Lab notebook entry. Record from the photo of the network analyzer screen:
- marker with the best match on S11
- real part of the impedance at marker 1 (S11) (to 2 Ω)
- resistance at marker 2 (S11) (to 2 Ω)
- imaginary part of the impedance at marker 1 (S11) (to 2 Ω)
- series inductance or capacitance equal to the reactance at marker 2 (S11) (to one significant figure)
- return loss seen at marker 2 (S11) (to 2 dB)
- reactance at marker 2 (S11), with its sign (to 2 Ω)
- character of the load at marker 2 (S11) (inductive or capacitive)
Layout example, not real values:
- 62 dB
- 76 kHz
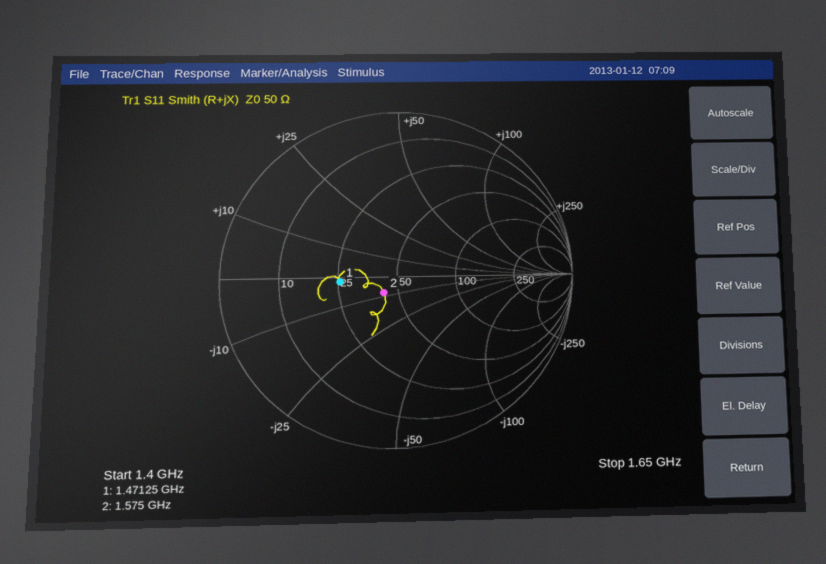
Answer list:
- marker 2
- 26 Ω
- 42 Ω
- -2 Ω
- 10 pF
- 18 dB
- -8 Ω
- capacitive
